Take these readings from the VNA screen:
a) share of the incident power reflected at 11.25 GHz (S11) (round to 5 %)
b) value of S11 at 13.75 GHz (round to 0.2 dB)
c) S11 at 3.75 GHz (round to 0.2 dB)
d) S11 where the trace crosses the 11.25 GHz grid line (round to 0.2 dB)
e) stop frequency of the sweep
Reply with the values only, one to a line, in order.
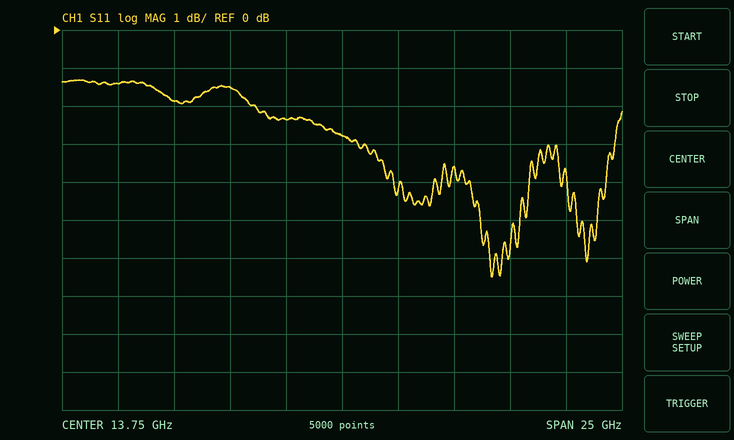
60 %
-2.8 dB
-1.4 dB
-2.4 dB
26.25 GHz
